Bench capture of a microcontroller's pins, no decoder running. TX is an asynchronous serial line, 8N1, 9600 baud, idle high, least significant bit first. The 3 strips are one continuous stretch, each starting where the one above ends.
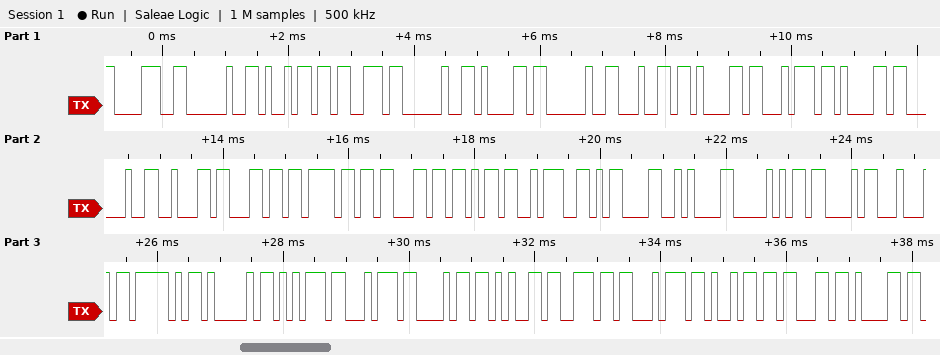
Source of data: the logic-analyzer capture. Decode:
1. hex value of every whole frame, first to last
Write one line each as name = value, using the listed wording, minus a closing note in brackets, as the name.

hex value of every whole frame, first to last = 38 20 69 73 20 61 20 64 61 74 61 20 62 6C 6F 63 6B 3A 0D 0A 50 43 44 5F 41 75 74 68 65 6E 74 69 63 61
